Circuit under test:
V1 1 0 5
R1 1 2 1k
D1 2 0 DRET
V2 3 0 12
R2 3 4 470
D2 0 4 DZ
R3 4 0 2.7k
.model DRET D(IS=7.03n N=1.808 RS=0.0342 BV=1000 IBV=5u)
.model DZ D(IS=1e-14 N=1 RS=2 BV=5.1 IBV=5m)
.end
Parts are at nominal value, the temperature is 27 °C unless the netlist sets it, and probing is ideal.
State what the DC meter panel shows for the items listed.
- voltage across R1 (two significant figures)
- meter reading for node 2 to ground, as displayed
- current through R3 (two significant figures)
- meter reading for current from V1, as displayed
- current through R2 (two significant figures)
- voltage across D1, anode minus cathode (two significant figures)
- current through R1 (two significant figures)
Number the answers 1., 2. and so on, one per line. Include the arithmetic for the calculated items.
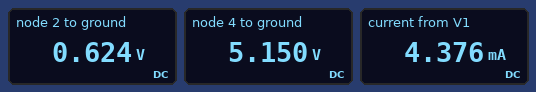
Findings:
1. 5 V - 624 mV = 4.4 V
2. 0.624 V
3. (5.15 V) / 2.7 kΩ = 1.9 mA
4. 4.376 mA
5. (12 V - 5.15 V) / 470 Ω = 15 mA
6. 624 mV = 620 mV
7. (5 V - 624 mV) / 1 kΩ = 4.4 mA
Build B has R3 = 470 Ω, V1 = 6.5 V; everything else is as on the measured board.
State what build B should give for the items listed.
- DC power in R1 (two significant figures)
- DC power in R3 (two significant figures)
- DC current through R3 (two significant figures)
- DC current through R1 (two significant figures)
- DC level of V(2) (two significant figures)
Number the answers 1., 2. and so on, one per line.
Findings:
1. 34 mW
2. 55 mW
3. 11 mA
4. 5.9 mA
5. 640 mV
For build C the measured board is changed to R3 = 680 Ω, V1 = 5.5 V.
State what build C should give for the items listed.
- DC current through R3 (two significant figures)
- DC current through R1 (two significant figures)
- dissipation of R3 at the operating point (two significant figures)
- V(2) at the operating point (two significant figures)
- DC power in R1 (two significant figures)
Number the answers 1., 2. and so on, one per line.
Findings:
1. 7.5 mA
2. 4.9 mA
3. 39 mW
4. 630 mV
5. 24 mW
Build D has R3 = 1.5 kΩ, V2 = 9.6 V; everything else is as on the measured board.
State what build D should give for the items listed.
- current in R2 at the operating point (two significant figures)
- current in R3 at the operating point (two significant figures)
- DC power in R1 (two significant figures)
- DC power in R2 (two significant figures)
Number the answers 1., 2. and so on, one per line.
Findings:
1. 9.5 mA
2. 3.4 mA
3. 19 mW
4. 43 mW
